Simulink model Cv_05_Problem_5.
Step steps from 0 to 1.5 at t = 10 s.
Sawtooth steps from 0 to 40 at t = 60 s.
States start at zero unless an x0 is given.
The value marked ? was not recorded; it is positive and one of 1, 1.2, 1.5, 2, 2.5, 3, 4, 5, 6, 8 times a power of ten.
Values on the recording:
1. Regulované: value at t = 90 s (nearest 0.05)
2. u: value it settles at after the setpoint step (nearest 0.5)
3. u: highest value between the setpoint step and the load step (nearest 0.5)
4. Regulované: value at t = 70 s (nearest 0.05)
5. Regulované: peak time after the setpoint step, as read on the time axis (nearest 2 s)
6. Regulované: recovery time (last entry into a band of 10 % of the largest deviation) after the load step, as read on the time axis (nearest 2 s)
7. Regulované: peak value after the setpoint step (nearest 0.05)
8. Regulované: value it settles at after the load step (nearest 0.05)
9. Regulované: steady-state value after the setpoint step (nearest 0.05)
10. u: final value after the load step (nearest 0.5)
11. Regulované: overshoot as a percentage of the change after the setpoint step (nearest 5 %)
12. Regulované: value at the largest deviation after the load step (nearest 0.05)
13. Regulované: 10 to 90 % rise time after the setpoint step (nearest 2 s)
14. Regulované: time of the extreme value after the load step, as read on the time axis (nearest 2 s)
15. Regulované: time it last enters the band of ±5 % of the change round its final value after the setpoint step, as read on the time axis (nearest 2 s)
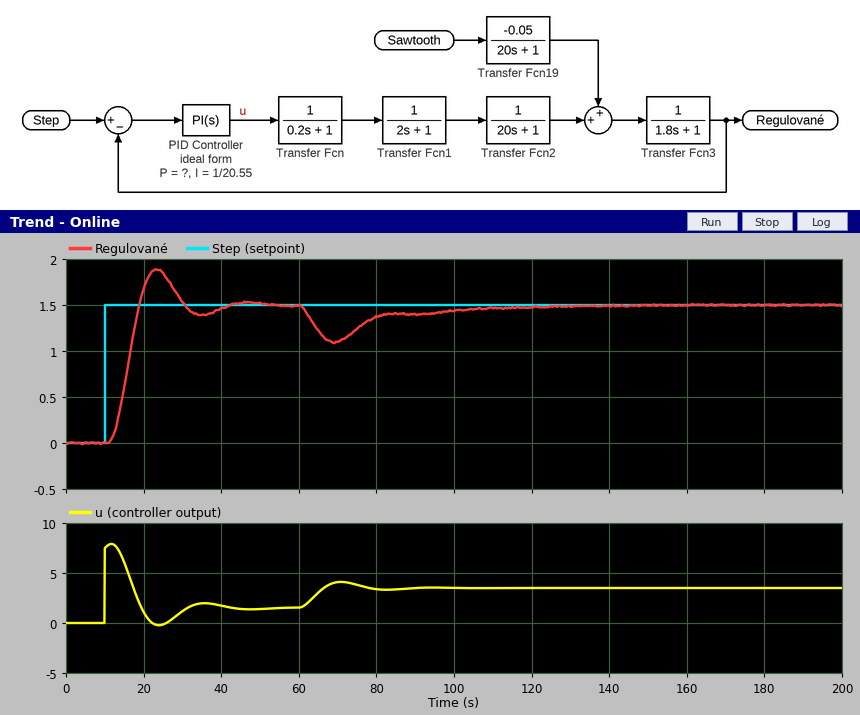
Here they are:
1.40
1.5
8.0
1.10
24 s
108 s
1.90
1.50
1.50
3.5
25 %
1.10
6 s
70 s
38 s
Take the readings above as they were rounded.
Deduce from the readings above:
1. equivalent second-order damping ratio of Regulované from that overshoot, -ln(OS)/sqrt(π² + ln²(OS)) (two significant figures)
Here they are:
0.40
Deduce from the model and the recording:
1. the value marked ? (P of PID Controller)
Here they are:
5
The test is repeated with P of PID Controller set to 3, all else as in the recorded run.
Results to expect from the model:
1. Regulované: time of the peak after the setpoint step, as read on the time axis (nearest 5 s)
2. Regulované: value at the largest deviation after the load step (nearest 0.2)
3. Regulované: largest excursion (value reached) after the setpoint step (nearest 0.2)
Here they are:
30 s
1.0
1.6
